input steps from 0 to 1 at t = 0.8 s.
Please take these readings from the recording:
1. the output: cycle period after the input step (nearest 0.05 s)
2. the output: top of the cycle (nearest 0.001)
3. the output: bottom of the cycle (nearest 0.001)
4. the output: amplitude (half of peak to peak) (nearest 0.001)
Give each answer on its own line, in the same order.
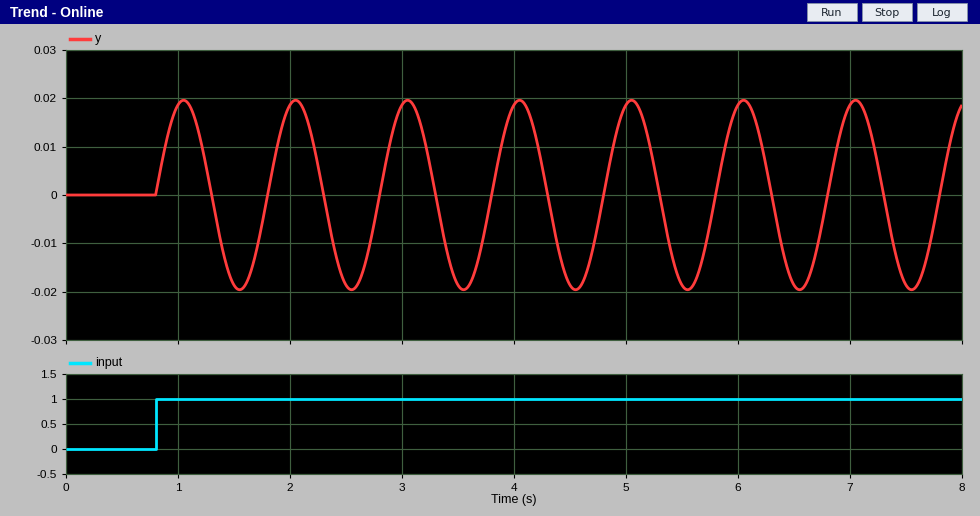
1.00 s
0.020
-0.020
0.020
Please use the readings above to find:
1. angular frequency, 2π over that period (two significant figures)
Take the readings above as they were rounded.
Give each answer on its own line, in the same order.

6.3 rad/s
